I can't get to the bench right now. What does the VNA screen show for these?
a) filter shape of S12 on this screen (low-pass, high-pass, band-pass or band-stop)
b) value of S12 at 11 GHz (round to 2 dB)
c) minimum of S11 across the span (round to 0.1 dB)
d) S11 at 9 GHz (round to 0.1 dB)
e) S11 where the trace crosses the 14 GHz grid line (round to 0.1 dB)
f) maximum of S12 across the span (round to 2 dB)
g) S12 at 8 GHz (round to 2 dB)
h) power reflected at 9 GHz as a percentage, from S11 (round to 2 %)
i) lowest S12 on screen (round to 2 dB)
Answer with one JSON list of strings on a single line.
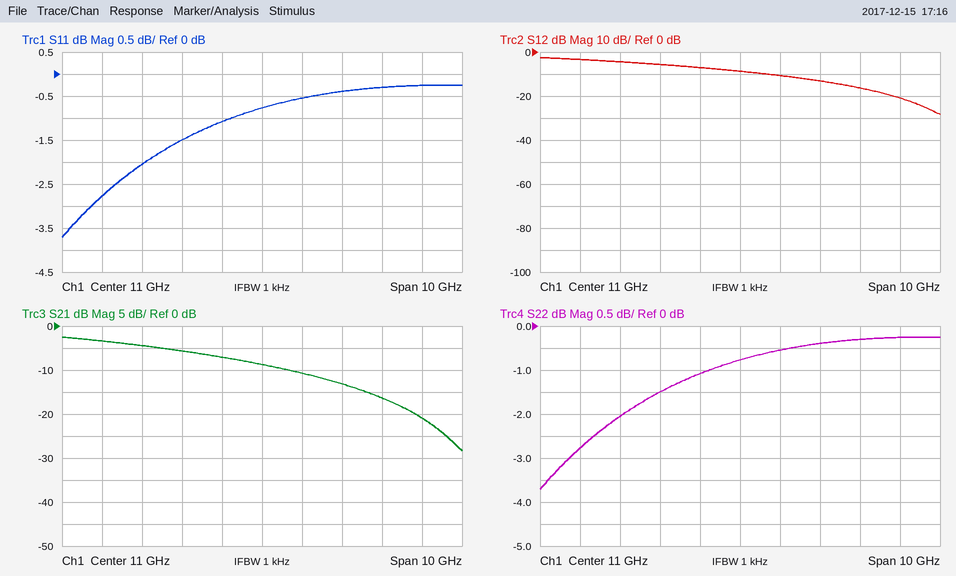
["low-pass", "-8 dB", "-3.7 dB", "-1.5 dB", "-0.3 dB", "-2 dB", "-4 dB", "70 %", "-28 dB"]
